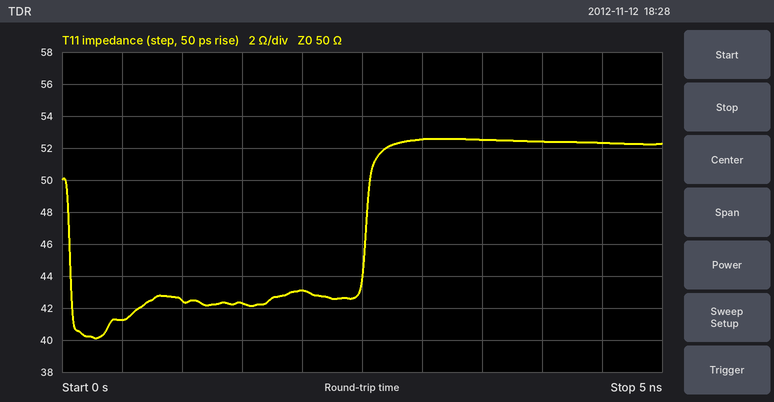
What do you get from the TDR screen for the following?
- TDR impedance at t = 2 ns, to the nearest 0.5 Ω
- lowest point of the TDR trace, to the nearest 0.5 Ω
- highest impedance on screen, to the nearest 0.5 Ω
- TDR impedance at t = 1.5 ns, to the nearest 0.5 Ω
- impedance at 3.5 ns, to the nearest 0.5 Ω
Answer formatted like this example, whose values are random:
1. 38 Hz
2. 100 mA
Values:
1. 43.0 Ω
2. 40.0 Ω
3. 52.5 Ω
4. 42.5 Ω
5. 52.5 Ω
